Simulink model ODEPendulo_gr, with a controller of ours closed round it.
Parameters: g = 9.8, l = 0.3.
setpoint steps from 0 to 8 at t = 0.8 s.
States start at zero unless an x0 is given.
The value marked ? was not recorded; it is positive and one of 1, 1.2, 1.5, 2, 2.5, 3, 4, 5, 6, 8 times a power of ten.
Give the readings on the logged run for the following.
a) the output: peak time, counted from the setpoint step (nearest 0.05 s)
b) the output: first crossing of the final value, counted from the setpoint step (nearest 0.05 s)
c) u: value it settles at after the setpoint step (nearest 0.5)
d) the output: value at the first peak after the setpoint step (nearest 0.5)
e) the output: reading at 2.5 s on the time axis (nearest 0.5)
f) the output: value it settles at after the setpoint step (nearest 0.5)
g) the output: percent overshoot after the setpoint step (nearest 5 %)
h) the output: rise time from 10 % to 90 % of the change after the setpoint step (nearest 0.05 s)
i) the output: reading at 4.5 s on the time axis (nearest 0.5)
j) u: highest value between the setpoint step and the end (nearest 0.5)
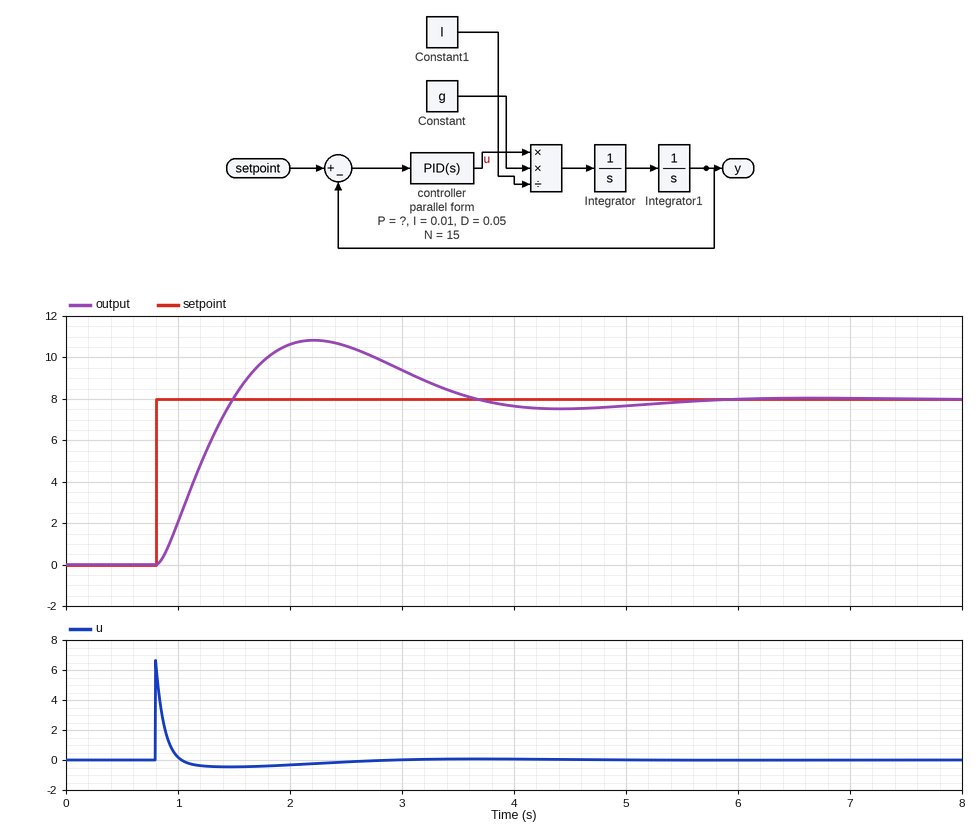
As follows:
1.40 s
0.70 s
0.0
11.0
10.5
8.0
35 %
0.50 s
7.5
6.5
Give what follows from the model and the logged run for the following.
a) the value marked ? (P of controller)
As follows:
0.08
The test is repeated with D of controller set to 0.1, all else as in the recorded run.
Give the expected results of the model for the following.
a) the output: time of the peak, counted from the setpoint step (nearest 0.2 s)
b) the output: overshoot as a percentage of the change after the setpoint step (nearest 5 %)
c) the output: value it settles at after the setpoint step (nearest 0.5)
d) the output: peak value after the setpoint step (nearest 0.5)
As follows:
1.0 s
15 %
8.0
9.5
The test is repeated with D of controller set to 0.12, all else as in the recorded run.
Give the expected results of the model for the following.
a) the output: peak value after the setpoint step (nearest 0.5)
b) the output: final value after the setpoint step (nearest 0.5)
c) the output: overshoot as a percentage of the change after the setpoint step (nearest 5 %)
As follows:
9.0
8.0
15 %
